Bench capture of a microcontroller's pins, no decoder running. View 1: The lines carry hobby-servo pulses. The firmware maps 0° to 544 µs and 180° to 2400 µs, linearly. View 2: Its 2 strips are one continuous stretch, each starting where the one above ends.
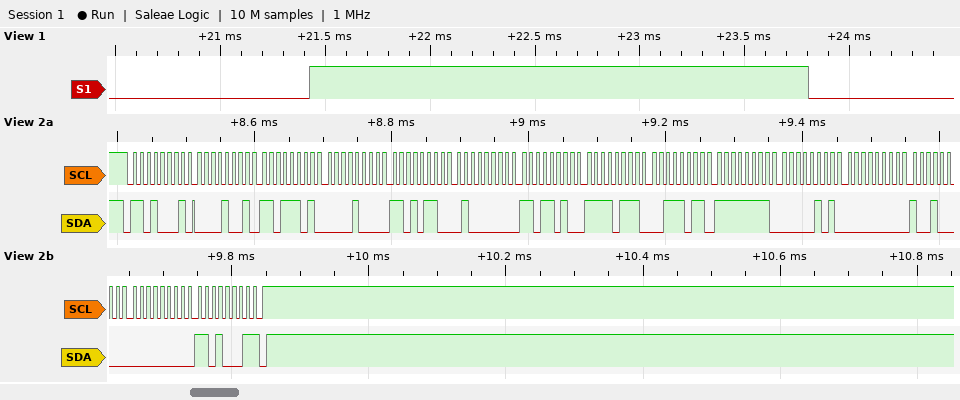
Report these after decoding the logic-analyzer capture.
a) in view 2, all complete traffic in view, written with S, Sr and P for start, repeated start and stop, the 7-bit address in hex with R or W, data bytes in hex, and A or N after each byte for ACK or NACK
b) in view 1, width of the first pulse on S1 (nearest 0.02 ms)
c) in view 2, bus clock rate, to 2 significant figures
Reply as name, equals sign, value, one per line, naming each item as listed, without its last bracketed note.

in view 2, all complete traffic in view, written with S, Sr and P for start, repeated start and stop, the 7-bit address in hex with R or W, data bytes in hex, and A or N after each byte for ACK or NACK = S 68R A 09 A DD A 08 A D6 A 40 A DA A F7 A 3B A FF A 05 A 00 A 90 A 00 A D1 N P
in view 1, width of the first pulse on S1 = 2.38 ms
in view 2, bus clock rate, to 2 significant figures = 100 kHz
